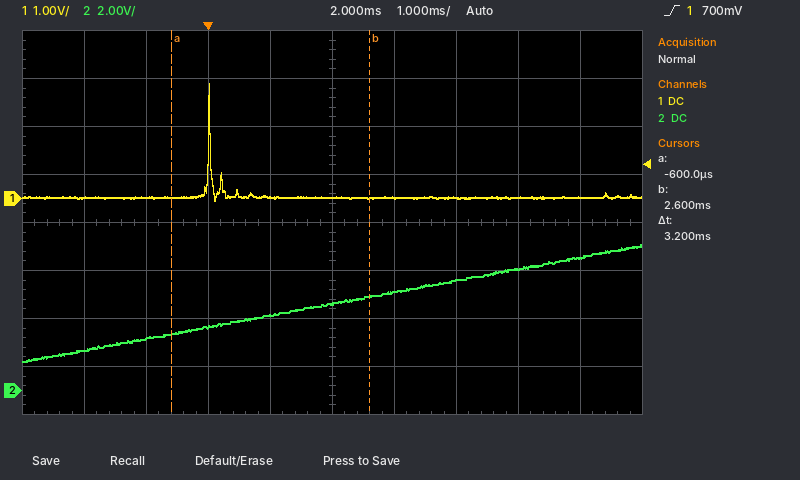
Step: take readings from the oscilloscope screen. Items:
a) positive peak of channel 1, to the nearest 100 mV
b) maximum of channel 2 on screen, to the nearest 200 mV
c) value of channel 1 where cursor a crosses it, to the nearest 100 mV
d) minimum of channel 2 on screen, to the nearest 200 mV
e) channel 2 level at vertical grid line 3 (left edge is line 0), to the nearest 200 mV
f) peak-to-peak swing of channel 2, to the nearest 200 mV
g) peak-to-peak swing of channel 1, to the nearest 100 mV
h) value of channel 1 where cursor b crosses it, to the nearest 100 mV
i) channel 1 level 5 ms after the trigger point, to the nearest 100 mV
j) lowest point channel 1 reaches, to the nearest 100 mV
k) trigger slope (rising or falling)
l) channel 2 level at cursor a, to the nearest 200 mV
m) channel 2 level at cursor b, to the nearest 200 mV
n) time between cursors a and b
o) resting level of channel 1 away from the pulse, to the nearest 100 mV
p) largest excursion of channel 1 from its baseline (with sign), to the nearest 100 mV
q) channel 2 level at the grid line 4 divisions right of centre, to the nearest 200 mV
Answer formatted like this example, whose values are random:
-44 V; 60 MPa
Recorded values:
2.4 V; 6.0 V; 0.0 V; 1.2 V; 2.6 V; 4.8 V; 2.4 V; 0.0 V; 0.0 V; 0.0 V; rising; 2.4 V; 4.0 V; 3.2 ms; 0.0 V; +2.4 V; 5.6 V
